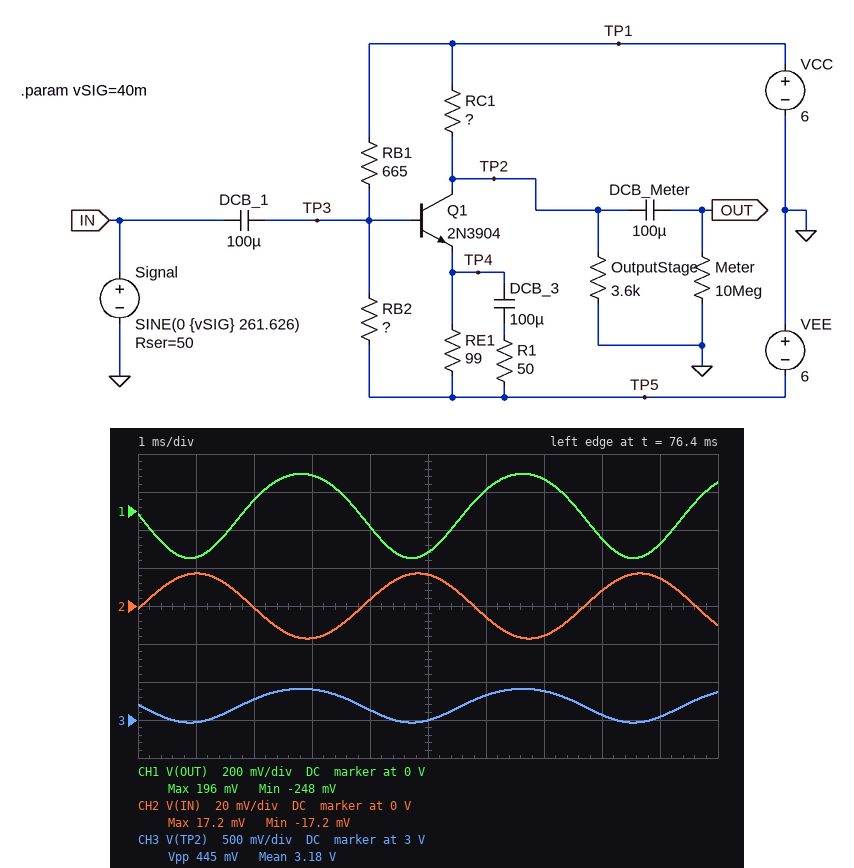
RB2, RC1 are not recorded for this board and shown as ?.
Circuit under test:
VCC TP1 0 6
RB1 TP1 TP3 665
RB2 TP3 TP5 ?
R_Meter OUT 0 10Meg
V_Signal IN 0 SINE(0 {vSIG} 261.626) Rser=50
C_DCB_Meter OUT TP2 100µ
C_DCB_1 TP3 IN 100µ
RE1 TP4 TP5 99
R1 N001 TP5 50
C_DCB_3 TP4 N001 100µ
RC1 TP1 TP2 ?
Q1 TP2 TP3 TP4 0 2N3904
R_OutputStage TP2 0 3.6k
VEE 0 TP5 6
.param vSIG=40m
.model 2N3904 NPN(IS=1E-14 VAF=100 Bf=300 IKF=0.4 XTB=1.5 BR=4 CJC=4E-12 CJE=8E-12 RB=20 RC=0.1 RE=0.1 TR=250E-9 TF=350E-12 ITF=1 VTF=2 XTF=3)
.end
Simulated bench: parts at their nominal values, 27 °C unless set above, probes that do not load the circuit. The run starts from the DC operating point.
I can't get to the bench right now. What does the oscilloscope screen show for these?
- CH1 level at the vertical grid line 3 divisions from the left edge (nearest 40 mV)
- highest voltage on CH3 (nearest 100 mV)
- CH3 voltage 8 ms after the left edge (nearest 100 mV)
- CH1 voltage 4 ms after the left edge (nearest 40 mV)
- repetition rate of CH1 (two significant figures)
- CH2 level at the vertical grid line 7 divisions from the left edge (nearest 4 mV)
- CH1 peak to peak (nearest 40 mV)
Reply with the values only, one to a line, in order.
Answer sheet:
200 mV
3.4 V
3.1 V
-80 mV
260 Hz
-16 mV
440 mV
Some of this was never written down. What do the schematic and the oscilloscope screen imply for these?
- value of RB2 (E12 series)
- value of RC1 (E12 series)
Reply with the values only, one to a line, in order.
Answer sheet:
39 Ω
2.2 kΩ
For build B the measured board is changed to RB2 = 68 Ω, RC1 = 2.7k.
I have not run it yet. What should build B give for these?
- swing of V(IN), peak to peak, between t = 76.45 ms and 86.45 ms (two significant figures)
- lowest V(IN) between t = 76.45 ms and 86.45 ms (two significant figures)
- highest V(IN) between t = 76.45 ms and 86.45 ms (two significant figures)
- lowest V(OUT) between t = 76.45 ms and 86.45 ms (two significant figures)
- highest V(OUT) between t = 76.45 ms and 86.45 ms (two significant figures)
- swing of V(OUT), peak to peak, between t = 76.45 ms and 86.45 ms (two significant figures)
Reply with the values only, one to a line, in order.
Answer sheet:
44 mV
-22 mV
22 mV
-850 mV
840 mV
1.7 V
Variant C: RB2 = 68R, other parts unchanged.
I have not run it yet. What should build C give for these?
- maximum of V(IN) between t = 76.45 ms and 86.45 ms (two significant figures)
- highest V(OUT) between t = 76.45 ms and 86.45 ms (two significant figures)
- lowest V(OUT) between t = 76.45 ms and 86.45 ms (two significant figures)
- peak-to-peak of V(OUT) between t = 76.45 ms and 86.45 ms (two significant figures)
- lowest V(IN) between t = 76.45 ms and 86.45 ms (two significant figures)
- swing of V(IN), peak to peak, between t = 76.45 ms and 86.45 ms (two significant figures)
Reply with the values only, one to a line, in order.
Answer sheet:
22 mV
740 mV
-750 mV
1.5 V
-22 mV
44 mV
